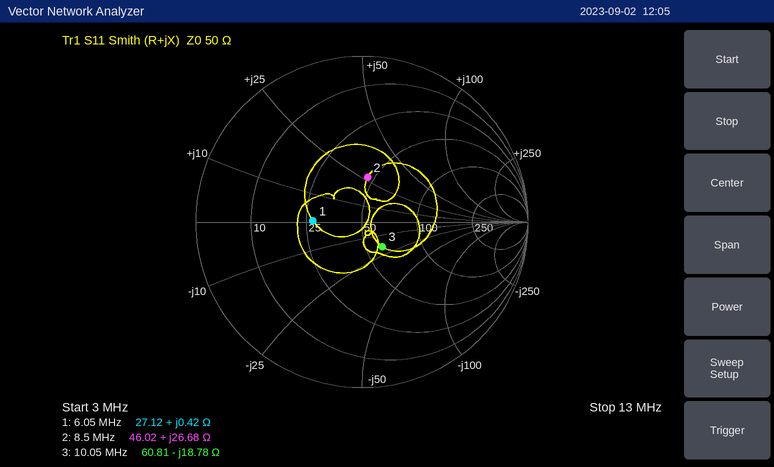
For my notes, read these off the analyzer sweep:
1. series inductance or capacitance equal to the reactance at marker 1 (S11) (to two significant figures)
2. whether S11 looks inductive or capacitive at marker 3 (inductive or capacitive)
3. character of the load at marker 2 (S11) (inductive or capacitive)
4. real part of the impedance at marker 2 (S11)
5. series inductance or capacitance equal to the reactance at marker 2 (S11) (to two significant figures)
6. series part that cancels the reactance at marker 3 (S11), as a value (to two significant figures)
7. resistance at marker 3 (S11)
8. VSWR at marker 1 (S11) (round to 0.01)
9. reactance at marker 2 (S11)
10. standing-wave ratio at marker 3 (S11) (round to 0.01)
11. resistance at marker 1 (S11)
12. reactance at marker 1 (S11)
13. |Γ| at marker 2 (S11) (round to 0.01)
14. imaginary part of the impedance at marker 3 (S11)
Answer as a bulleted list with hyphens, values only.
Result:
- 11 nH
- capacitive
- inductive
- 46.02 Ω
- 500 nH
- 300 nH
- 60.81 Ω
- 1.84
- +26.68 Ω
- 1.48
- 27.12 Ω
- +0.42 Ω
- 0.27
- -18.78 Ω
